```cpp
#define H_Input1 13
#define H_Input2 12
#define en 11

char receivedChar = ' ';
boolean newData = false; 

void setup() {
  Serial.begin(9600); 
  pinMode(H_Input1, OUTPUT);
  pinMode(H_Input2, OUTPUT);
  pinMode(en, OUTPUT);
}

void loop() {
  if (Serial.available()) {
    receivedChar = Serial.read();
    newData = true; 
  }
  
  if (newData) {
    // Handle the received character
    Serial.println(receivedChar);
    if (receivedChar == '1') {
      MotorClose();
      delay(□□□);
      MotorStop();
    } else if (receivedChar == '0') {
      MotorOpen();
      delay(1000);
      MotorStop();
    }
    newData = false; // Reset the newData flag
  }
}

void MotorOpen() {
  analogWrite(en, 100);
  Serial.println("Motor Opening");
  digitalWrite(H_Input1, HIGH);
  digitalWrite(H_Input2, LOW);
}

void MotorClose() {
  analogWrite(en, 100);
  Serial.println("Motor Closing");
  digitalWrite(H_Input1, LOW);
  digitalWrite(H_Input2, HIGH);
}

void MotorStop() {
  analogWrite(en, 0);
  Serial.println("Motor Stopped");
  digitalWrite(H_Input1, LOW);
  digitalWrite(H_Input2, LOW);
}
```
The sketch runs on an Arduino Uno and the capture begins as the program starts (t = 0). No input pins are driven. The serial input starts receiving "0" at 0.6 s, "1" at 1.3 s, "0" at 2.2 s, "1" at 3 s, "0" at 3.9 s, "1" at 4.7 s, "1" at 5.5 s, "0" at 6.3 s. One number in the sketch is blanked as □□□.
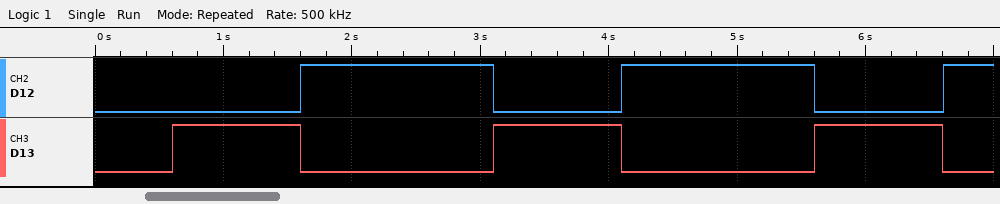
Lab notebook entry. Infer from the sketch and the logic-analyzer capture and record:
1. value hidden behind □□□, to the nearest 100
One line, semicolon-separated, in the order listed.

1500
